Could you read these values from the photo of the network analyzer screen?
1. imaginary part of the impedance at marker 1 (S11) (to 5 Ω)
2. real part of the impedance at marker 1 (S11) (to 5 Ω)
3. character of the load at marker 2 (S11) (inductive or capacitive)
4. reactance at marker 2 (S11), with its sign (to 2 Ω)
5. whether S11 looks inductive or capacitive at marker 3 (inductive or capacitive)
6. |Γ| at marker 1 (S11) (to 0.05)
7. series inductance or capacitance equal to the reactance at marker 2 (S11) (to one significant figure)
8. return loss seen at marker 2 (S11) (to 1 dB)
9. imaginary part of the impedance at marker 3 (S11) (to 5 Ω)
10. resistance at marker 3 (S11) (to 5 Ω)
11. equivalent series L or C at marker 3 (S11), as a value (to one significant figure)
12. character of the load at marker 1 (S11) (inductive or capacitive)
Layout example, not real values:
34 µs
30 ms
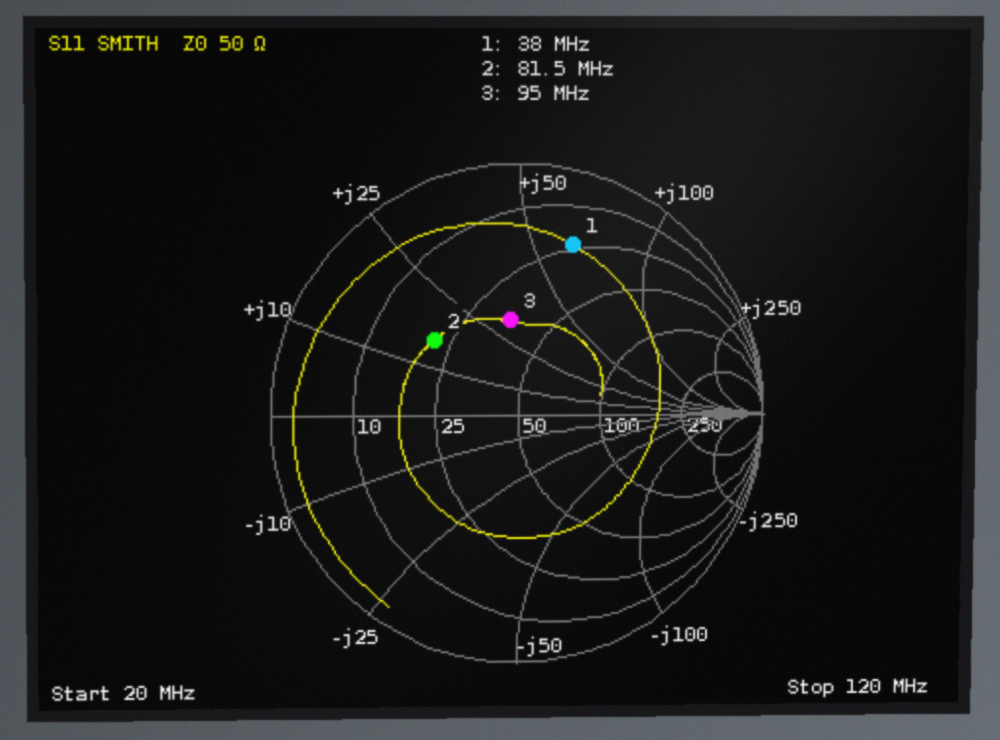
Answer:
+65 Ω
25 Ω
inductive
+16 Ω
inductive
0.70
30 nH
7 dB
+30 Ω
35 Ω
50 nH
inductive
